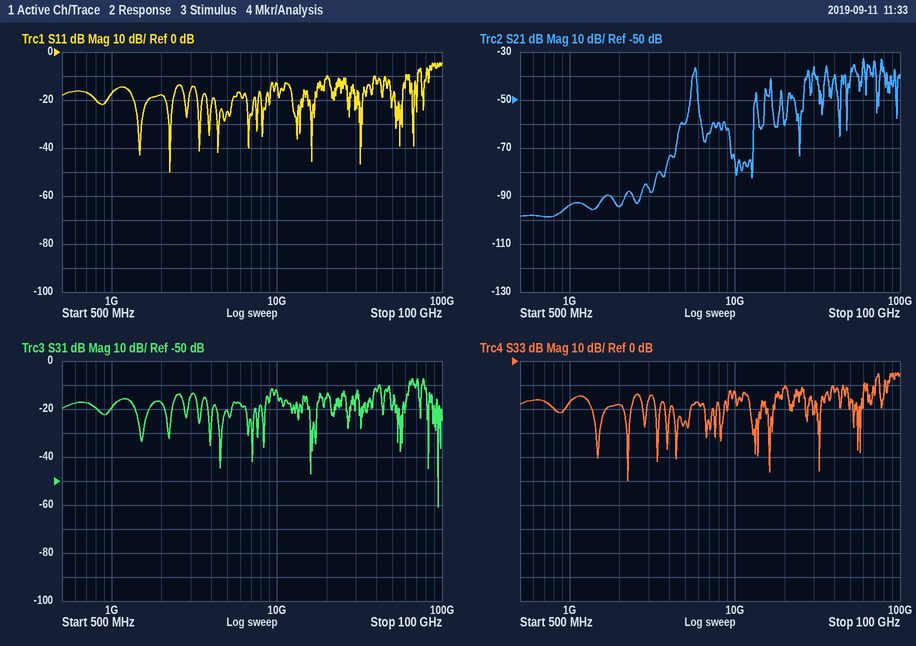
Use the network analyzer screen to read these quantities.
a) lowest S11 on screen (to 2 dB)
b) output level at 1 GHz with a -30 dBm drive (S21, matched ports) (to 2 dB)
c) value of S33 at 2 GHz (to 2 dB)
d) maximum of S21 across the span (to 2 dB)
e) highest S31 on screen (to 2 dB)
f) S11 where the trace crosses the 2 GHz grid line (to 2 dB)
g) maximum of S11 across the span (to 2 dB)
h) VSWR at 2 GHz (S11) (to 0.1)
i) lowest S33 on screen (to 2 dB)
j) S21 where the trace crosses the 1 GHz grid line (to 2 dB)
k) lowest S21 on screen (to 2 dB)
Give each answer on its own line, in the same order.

-50 dB
-124 dBm
-18 dB
-32 dB
-8 dB
-18 dB
-4 dB
1.3
-50 dB
-94 dB
-98 dB
